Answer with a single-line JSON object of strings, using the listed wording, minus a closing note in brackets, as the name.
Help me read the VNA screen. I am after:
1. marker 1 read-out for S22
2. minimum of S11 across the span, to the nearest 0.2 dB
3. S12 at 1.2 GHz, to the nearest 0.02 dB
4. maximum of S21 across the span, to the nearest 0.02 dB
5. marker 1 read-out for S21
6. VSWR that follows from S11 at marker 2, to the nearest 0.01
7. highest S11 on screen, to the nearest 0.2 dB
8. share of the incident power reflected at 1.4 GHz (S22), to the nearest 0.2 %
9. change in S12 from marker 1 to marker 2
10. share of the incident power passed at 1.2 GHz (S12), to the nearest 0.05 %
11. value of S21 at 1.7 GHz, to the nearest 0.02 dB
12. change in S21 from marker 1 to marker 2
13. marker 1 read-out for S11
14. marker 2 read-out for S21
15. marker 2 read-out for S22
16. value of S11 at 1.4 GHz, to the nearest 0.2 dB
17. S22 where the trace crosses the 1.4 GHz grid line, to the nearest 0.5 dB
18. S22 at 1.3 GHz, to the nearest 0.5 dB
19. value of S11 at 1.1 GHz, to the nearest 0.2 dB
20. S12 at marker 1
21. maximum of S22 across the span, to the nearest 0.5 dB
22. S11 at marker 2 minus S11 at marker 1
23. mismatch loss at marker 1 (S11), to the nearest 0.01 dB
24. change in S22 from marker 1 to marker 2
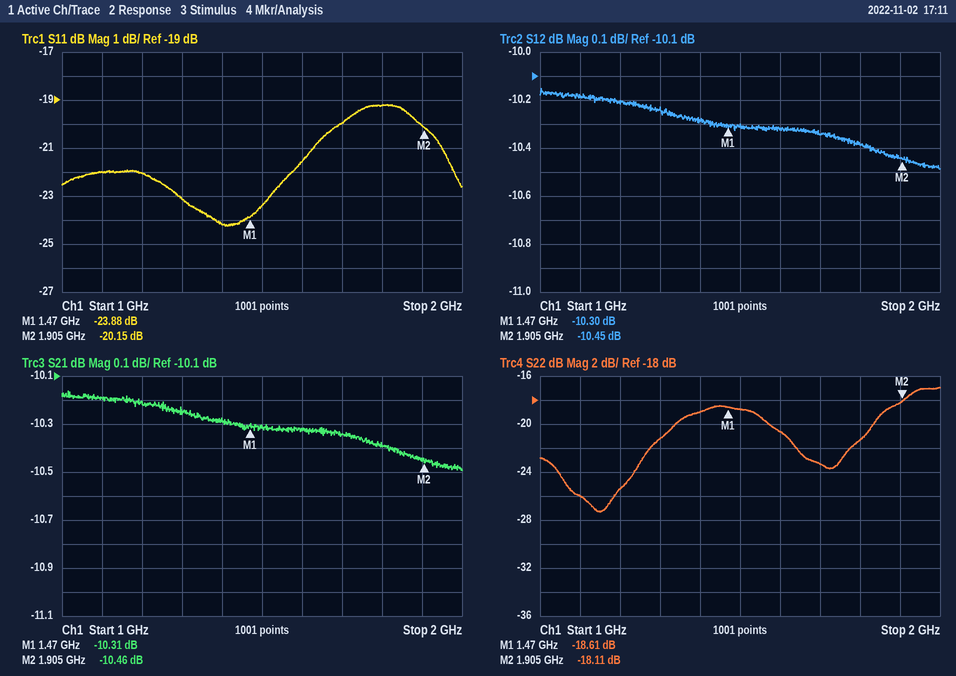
{"marker 1 read-out for S22": "-18.61 dB", "minimum of S11 across the span, to the nearest 0.2 dB": "-24.2 dB", "S12 at 1.2 GHz, to the nearest 0.02 dB": "-10.20 dB", "maximum of S21 across the span, to the nearest 0.02 dB": "-10.16 dB", "marker 1 read-out for S21": "-10.31 dB", "VSWR that follows from S11 at marker 2, to the nearest 0.01": "1.22", "highest S11 on screen, to the nearest 0.2 dB": "-19.2 dB", "share of the incident power reflected at 1.4 GHz (S22), to the nearest 0.2 %": "1.2 %", "change in S12 from marker 1 to marker 2": "-0.15 dB", "share of the incident power passed at 1.2 GHz (S12), to the nearest 0.05 %": "9.55 %", "value of S21 at 1.7 GHz, to the nearest 0.02 dB": "-10.34 dB", "change in S21 from marker 1 to marker 2": "-0.15 dB", "marker 1 read-out for S11": "-23.88 dB", "marker 2 read-out for S21": "-10.46 dB", "marker 2 read-out for S22": "-18.11 dB", "value of S11 at 1.4 GHz, to the nearest 0.2 dB": "-24.2 dB", "S22 where the trace crosses the 1.4 GHz grid line, to the nearest 0.5 dB": "-19.0 dB", "S22 at 1.3 GHz, to the nearest 0.5 dB": "-21.0 dB", "value of S11 at 1.1 GHz, to the nearest 0.2 dB": "-22.0 dB", "S12 at marker 1": "-10.30 dB", "maximum of S22 across the span, to the nearest 0.5 dB": "-17.0 dB", "S11 at marker 2 minus S11 at marker 1": "3.73 dB", "mismatch loss at marker 1 (S11), to the nearest 0.01 dB": "0.02 dB", "change in S22 from marker 1 to marker 2": "0.50 dB"}
